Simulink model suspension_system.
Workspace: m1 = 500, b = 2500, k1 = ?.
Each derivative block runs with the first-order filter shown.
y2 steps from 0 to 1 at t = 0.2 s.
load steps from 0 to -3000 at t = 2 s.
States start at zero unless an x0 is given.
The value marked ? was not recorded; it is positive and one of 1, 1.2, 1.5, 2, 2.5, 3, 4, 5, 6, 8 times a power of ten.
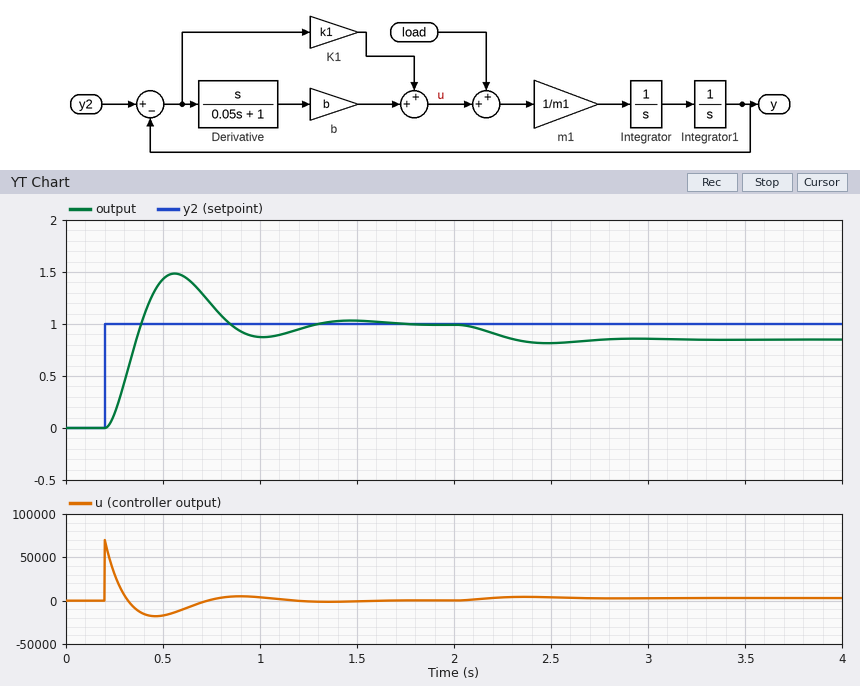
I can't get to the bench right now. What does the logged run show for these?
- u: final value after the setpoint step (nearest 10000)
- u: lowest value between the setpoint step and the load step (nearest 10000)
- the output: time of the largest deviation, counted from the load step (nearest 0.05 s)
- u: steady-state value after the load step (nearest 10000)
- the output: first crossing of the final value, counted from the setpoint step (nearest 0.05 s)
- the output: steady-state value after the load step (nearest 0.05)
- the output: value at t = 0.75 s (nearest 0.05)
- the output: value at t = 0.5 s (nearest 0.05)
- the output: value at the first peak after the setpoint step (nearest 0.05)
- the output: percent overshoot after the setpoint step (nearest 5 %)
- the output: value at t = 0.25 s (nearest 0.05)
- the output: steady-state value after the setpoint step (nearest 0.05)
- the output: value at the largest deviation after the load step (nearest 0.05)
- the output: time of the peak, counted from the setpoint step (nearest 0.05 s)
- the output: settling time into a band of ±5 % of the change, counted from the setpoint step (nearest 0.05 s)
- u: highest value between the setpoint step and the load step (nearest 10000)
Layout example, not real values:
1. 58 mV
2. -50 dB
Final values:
1. 0
2. -20000
3. 0.50 s
4. 0
5. 0.20 s
6. 0.85
7. 1.20
8. 1.45
9. 1.50
10. 50 %
11. 0.15
12. 1.00
13. 0.80
14. 0.35 s
15. 1.00 s
16. 70000
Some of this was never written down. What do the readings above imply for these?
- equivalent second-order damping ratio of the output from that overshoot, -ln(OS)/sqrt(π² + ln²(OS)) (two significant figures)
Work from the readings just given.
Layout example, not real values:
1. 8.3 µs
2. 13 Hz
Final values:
1. 0.22
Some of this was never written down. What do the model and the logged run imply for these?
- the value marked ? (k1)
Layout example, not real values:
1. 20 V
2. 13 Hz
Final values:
1. 20000
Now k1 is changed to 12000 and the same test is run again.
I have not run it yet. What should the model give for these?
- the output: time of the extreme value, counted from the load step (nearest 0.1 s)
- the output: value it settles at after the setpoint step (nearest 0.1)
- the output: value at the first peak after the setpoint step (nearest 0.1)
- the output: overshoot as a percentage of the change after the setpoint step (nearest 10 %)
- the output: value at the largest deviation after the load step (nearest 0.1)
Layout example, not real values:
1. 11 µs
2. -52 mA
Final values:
1. 0.7 s
2. 1.0
3. 1.4
4. 40 %
5. 0.7
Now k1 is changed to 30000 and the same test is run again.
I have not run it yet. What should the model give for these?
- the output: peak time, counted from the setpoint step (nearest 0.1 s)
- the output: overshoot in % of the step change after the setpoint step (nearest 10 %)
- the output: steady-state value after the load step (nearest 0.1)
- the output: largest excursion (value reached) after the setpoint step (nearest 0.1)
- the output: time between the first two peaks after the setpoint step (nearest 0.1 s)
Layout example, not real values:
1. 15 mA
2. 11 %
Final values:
1. 0.3 s
2. 60 %
3. 0.9
4. 1.6
5. 0.7 s
